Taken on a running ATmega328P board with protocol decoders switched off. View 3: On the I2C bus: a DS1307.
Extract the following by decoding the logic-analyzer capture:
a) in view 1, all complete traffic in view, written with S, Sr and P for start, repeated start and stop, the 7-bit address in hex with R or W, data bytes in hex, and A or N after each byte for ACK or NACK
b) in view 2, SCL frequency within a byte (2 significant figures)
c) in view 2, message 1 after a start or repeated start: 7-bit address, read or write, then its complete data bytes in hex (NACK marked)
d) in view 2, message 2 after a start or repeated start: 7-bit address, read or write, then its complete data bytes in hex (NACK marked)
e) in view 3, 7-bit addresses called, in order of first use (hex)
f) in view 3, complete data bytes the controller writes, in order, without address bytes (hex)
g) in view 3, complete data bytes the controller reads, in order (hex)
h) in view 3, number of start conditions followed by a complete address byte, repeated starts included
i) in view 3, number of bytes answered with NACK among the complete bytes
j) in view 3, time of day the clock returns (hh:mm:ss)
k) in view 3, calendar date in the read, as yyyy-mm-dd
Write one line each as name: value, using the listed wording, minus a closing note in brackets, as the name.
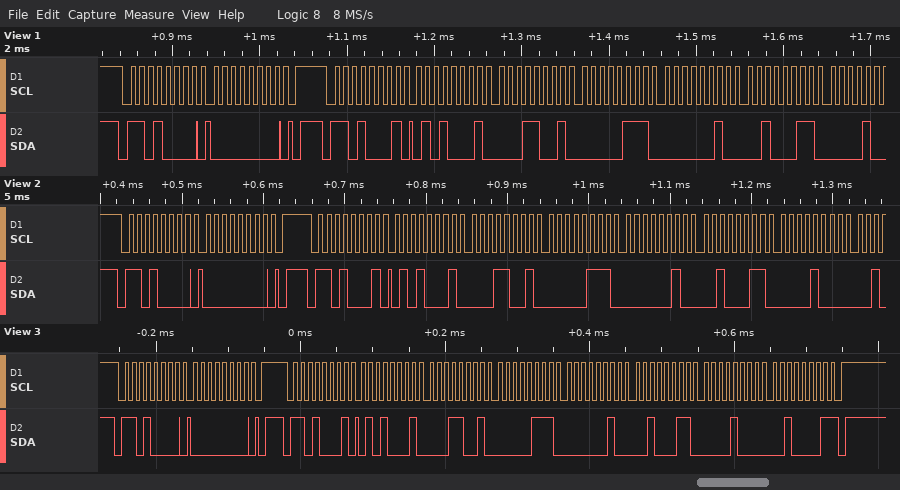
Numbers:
in view 1, all complete traffic in view, written with S, Sr and P for start, repeated start and stop, the 7-bit address in hex with R or W, data bytes in hex, and A or N after each byte for ACK or NACK: S 68W A 00 A P S 68R A 51 A 19 A 07 A 02 A 23 A
in view 2, SCL frequency within a byte: 100 kHz
in view 2, message 1 after a start or repeated start: 7-bit address, read or write, then its complete data bytes in hex: 0x68 write: 00
in view 2, message 2 after a start or repeated start: 7-bit address, read or write, then its complete data bytes in hex: 0x68 read: 51 19 07 02 23 08
in view 3, 7-bit addresses called, in order of first use: 0x68
in view 3, complete data bytes the controller writes, in order, without address bytes: 00
in view 3, complete data bytes the controller reads, in order: 51 19 07 02 23 08 21
in view 3, number of start conditions followed by a complete address byte, repeated starts included: 2
in view 3, number of bytes answered with NACK among the complete bytes: 1
in view 3, time of day the clock returns: 07:19:51
in view 3, calendar date in the read, as yyyy-mm-dd: 2021-08-23
